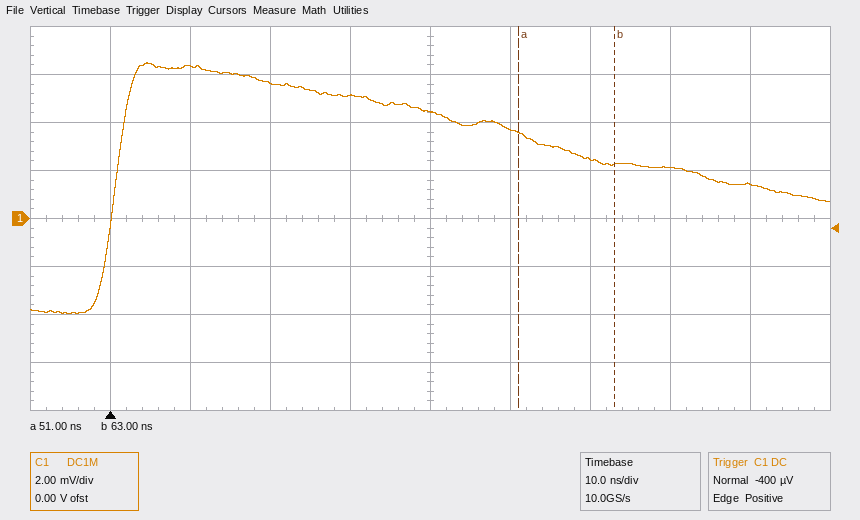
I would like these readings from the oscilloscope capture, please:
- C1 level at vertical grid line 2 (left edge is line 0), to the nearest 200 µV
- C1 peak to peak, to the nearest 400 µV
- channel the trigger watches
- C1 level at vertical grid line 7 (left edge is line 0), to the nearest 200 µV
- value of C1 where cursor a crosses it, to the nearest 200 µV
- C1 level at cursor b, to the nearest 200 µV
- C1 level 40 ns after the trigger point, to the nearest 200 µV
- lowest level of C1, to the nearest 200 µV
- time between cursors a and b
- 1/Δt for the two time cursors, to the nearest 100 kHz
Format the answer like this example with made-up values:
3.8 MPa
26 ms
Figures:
6.4 mV
10.4 mV
C1
2.4 mV
3.6 mV
2.2 mV
4.4 mV
-4.0 mV
12 ns
83.3 MHz
